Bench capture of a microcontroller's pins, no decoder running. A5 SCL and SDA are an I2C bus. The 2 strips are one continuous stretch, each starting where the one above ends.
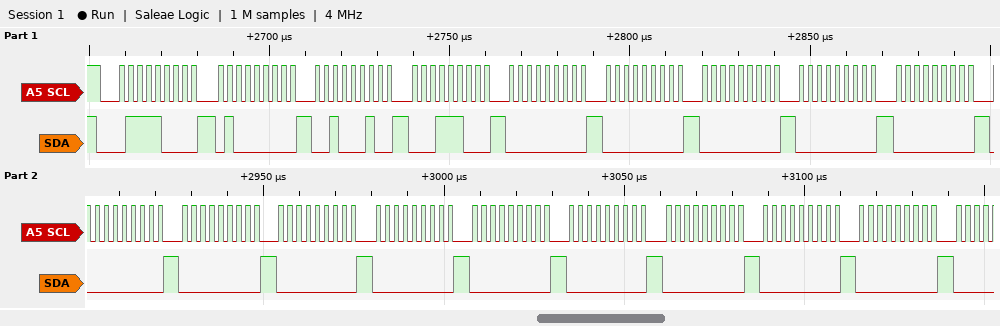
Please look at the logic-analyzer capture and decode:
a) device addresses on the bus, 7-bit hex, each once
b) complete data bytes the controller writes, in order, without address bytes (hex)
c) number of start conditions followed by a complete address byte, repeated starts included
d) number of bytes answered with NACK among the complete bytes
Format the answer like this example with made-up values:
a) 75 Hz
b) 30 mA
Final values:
a) 0x3C
b) 40 22 1C 00 00 00 00 00 00 00 00 00 00 00 00 00 00
c) 1
d) 0
